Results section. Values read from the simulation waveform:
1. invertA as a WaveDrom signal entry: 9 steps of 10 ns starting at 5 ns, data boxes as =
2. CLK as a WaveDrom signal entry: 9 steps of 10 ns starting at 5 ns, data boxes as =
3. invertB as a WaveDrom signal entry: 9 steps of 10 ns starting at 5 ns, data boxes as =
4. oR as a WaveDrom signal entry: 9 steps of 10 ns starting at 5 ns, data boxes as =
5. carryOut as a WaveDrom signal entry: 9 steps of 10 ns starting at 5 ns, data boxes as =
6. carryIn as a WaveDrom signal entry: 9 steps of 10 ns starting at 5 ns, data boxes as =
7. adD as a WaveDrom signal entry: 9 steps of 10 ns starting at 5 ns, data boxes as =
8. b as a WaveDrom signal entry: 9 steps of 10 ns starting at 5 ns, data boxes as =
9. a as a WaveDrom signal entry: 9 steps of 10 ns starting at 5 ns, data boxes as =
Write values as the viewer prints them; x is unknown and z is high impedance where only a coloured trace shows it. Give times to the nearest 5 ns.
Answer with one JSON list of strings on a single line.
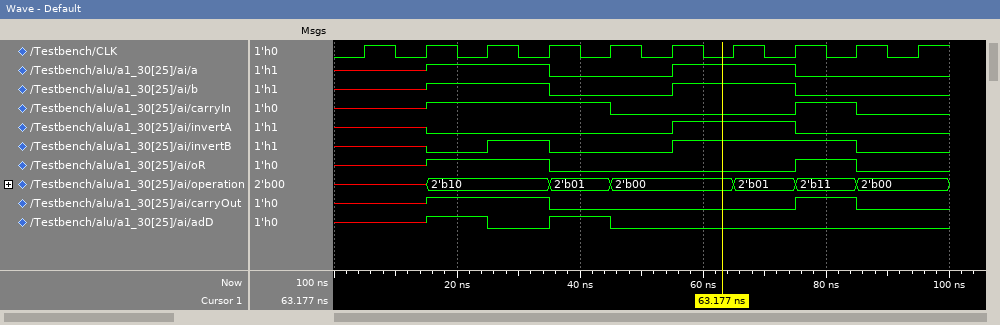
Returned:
["{name: 'invertA', wave: 'x0...1.0.'}", "{name: 'CLK', wave: 'p........'}", "{name: 'invertB', wave: 'x010.1..0'}", "{name: 'oR', wave: 'x1.0...10'}", "{name: 'carryOut', wave: 'x1.0...10'}", "{name: 'carryIn', wave: 'x1..0..10'}", "{name: 'adD', wave: 'x1010....'}", "{name: 'b', wave: 'x1.0.1.0.'}", "{name: 'a', wave: 'x1.0.1.0.'}"]
